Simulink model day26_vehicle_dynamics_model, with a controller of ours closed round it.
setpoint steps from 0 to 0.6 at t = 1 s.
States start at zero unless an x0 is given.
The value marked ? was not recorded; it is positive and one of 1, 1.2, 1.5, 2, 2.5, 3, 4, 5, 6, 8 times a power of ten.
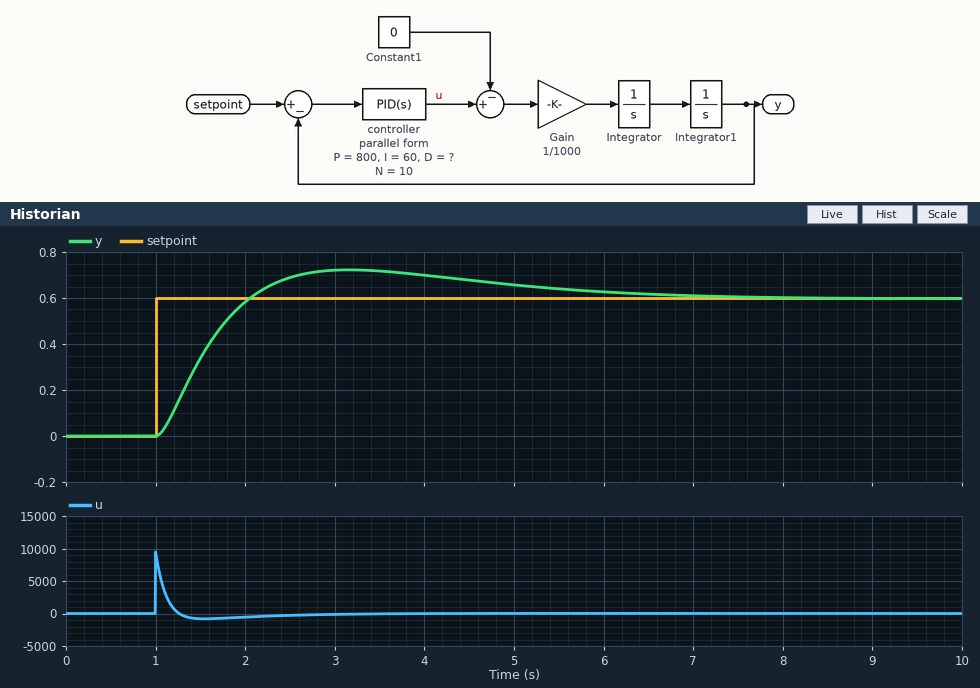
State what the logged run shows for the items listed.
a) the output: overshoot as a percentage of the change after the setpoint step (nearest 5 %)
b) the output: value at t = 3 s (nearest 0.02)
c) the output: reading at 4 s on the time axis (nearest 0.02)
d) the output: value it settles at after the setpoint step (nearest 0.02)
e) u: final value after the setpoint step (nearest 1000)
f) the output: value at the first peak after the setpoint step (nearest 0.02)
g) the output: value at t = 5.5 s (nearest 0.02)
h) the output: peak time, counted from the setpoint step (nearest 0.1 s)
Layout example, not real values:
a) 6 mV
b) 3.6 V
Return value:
a) 20 %
b) 0.72
c) 0.70
d) 0.60
e) 0
f) 0.72
g) 0.64
h) 2.2 s
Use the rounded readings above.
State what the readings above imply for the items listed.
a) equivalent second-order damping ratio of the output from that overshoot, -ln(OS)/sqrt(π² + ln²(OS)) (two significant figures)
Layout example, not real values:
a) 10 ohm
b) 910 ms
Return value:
a) 0.46
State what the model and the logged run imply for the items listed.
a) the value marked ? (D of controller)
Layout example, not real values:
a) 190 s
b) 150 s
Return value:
a) 1500
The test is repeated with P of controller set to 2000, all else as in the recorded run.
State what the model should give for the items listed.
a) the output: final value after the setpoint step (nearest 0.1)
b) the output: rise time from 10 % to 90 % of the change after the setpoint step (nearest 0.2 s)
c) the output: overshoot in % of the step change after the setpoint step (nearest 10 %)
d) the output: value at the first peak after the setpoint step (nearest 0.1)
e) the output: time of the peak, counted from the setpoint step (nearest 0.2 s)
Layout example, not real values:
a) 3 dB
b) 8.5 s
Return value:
a) 0.6
b) 0.6 s
c) 30 %
d) 0.8
e) 1.6 s
